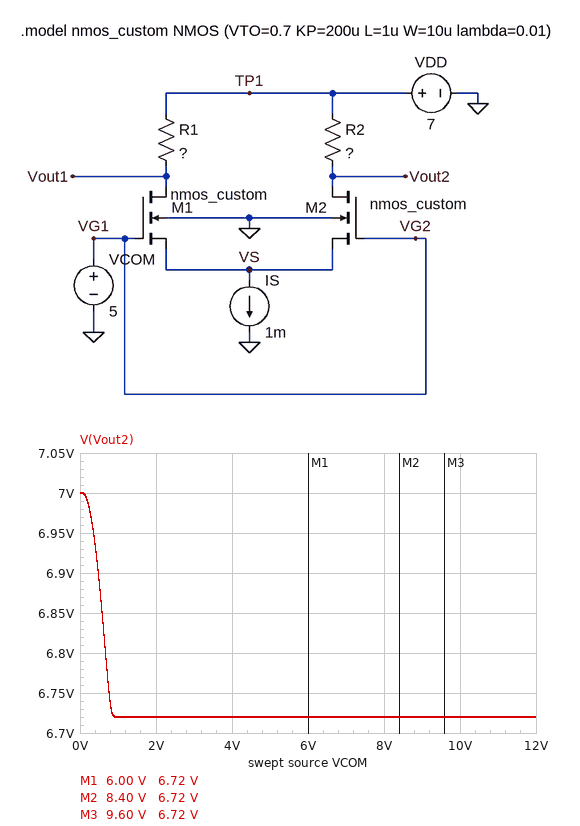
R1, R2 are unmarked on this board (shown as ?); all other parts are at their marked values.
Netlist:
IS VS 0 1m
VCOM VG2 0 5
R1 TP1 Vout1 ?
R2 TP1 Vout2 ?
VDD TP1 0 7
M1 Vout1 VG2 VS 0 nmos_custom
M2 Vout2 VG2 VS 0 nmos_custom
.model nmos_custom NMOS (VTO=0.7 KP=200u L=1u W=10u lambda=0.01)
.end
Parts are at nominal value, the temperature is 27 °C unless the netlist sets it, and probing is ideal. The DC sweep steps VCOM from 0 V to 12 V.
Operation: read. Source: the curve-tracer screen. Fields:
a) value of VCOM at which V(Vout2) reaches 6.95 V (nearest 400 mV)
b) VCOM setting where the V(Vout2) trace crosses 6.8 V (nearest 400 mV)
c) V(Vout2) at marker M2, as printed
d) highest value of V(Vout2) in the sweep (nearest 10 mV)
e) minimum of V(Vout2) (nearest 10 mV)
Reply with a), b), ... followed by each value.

a) 400 mV
b) 800 mV
c) 6.72 V
d) 7.00 V
e) 6.72 V
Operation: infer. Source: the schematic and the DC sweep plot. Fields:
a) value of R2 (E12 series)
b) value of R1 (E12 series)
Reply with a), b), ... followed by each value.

a) 560 Ω
b) 560 Ω
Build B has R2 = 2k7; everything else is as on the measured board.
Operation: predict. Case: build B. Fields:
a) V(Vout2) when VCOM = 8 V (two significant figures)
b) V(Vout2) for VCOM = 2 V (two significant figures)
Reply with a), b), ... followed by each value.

a) 6.3 V
b) 5.7 V
